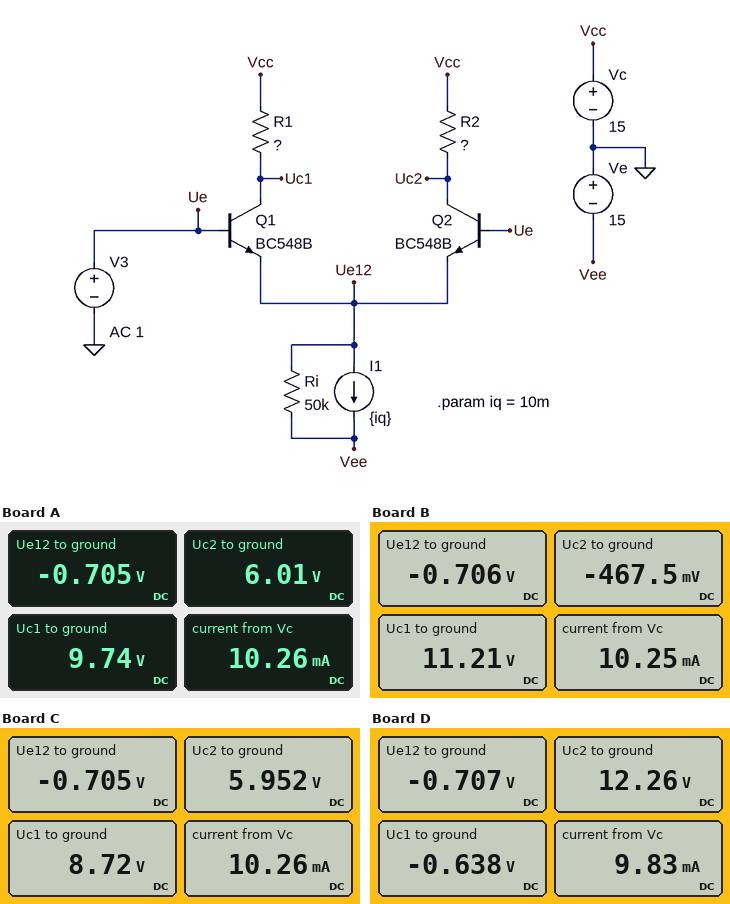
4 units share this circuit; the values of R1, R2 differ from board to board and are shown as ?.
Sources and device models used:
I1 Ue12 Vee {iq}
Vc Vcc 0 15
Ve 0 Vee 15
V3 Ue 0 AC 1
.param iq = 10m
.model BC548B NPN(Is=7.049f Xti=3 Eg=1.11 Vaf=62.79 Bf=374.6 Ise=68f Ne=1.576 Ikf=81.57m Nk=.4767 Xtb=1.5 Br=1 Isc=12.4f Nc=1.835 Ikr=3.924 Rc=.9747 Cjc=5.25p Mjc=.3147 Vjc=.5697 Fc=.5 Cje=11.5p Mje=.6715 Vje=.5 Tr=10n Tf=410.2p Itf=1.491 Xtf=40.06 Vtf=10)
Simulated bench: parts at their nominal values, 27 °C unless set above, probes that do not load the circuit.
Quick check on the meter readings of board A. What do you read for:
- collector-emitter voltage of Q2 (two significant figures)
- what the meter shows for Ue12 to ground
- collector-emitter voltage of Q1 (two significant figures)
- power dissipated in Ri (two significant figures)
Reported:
6.7 V
-0.705 V
10 V
4.1 mW
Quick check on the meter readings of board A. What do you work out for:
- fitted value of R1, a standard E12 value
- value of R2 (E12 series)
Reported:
1 kΩ
1.8 kΩ
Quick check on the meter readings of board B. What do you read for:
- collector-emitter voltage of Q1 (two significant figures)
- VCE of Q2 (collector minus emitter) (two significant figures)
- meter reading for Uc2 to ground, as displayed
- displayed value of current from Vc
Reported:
12 V
240 mV
-467.5 mV
10.25 mA
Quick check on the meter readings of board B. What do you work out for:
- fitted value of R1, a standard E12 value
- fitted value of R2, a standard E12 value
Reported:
680 Ω
3.3 kΩ
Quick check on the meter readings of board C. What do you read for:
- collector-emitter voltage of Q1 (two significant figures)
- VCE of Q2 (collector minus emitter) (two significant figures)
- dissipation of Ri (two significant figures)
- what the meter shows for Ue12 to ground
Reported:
9.4 V
6.7 V
4.1 mW
-0.705 V
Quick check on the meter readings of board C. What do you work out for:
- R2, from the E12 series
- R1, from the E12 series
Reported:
1.8 kΩ
1.2 kΩ
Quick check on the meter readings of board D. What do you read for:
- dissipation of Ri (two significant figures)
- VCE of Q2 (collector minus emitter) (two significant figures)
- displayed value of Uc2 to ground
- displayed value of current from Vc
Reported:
4.1 mW
13 V
12.26 V
9.83 mA
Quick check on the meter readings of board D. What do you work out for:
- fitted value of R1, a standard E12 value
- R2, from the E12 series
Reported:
3.9 kΩ
470 Ω
